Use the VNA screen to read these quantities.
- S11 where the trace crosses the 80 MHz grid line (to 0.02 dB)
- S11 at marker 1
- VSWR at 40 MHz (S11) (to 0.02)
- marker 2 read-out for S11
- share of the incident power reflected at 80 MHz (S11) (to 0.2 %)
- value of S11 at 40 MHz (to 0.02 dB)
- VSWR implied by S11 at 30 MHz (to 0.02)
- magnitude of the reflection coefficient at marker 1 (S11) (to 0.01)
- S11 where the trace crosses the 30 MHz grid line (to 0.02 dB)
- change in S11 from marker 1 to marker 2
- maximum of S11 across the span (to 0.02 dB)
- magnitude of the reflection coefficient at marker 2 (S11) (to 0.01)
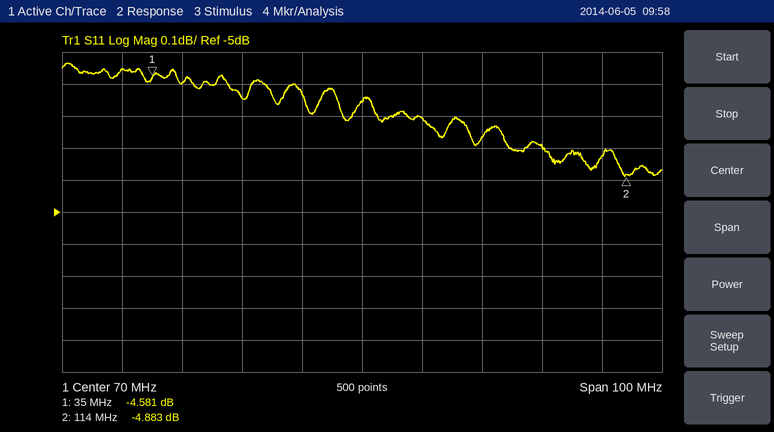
-4.70 dB
-4.581 dB
3.86
-4.883 dB
33.8 %
-4.60 dB
3.90
0.59
-4.56 dB
-0.302 dB
-4.54 dB
0.57
